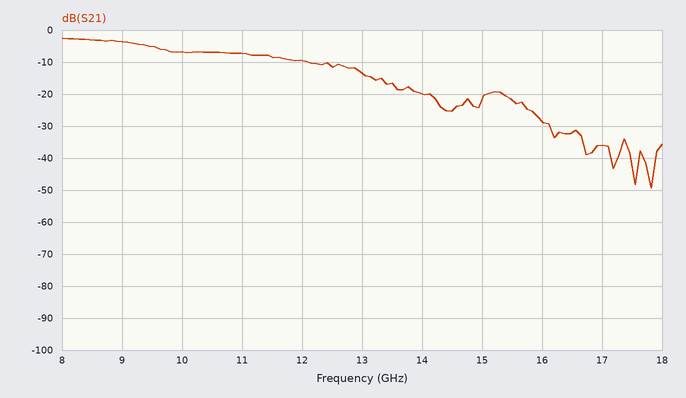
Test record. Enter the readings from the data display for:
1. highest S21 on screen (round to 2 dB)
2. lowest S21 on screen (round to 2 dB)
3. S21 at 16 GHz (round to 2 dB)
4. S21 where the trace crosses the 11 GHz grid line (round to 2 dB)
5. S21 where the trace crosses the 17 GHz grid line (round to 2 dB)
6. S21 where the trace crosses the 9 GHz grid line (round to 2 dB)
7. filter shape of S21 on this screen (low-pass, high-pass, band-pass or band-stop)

-2 dB
-50 dB
-28 dB
-8 dB
-36 dB
-4 dB
low-pass
